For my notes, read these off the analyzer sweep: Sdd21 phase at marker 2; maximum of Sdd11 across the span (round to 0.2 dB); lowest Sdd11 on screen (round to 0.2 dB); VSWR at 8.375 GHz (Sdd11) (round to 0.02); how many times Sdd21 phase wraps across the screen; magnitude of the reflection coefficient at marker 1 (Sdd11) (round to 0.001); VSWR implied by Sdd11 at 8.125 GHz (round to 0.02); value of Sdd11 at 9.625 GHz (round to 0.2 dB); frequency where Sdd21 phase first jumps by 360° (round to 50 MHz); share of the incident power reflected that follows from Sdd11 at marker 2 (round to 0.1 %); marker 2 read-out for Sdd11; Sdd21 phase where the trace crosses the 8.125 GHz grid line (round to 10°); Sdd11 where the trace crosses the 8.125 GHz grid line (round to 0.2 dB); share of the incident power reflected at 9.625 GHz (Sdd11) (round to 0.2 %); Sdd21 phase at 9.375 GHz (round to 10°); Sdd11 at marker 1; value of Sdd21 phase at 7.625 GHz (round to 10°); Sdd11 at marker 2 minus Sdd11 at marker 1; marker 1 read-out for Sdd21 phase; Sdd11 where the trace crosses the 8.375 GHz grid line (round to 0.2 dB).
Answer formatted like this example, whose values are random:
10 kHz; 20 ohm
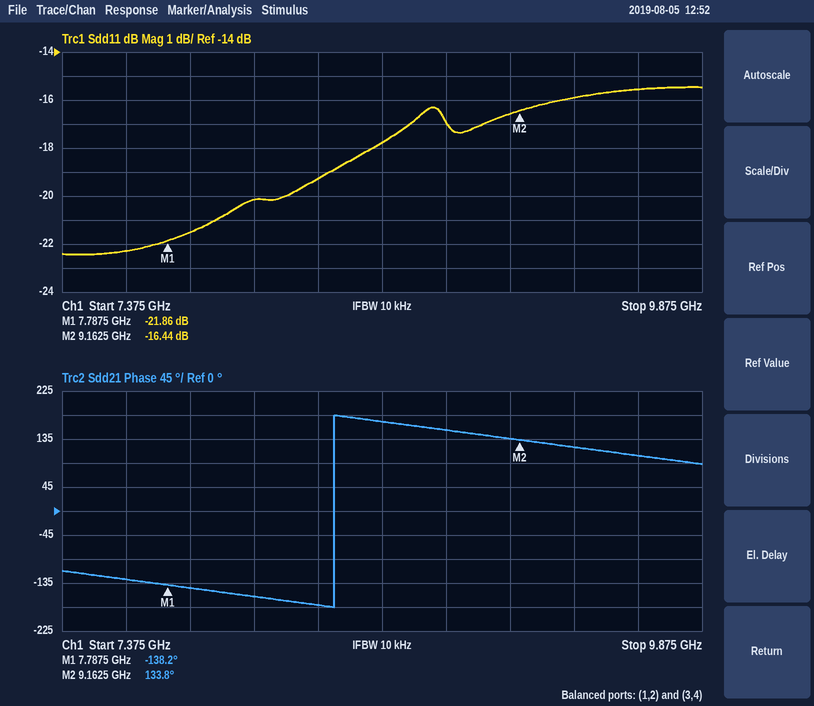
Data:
133.8°; -15.4 dB; -22.4 dB; 1.24; 1; 0.081; 1.22; -15.6 dB; 8.45 GHz; 2.3 %; -16.44 dB; -160°; -20.2 dB; 2.8 %; 120°; -21.86 dB; -130°; 5.42 dB; -138.2°; -19.2 dB
